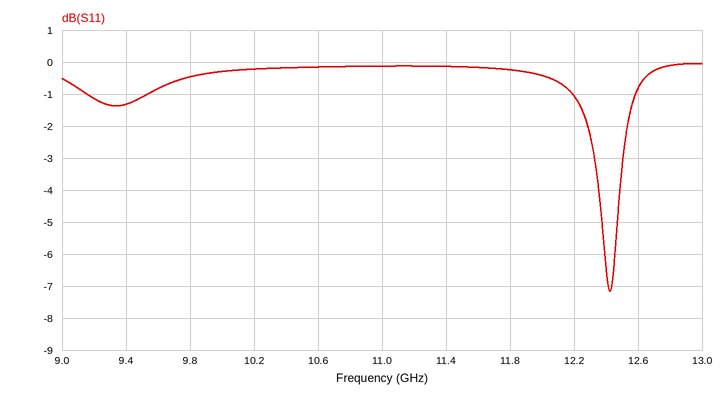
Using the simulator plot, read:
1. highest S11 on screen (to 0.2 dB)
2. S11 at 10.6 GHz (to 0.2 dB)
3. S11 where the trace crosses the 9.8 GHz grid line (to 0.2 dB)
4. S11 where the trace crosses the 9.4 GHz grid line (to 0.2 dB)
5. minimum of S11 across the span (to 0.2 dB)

0.0 dB
-0.2 dB
-0.4 dB
-1.4 dB
-7.2 dB
